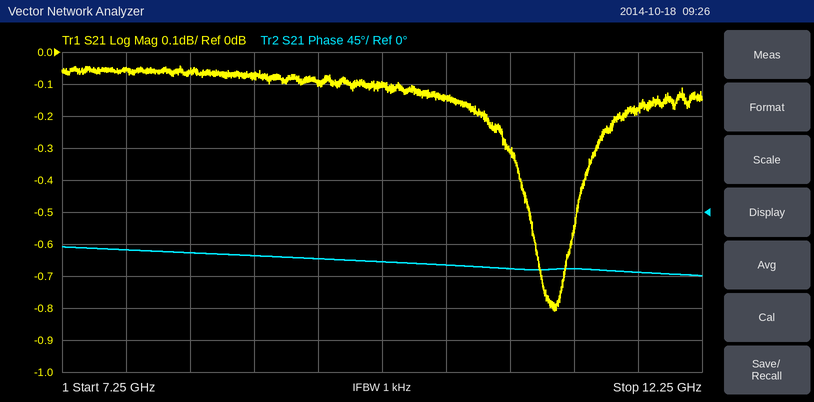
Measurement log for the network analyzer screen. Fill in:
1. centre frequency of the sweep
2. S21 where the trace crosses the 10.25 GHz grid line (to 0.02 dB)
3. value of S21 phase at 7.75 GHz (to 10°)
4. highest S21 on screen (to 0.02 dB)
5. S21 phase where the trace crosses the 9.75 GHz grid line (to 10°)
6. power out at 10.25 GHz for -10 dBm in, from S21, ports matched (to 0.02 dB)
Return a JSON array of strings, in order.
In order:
["9.75 GHz", "-0.14 dB", "-50°", "-0.04 dB", "-70°", "-10.14 dBm"]
